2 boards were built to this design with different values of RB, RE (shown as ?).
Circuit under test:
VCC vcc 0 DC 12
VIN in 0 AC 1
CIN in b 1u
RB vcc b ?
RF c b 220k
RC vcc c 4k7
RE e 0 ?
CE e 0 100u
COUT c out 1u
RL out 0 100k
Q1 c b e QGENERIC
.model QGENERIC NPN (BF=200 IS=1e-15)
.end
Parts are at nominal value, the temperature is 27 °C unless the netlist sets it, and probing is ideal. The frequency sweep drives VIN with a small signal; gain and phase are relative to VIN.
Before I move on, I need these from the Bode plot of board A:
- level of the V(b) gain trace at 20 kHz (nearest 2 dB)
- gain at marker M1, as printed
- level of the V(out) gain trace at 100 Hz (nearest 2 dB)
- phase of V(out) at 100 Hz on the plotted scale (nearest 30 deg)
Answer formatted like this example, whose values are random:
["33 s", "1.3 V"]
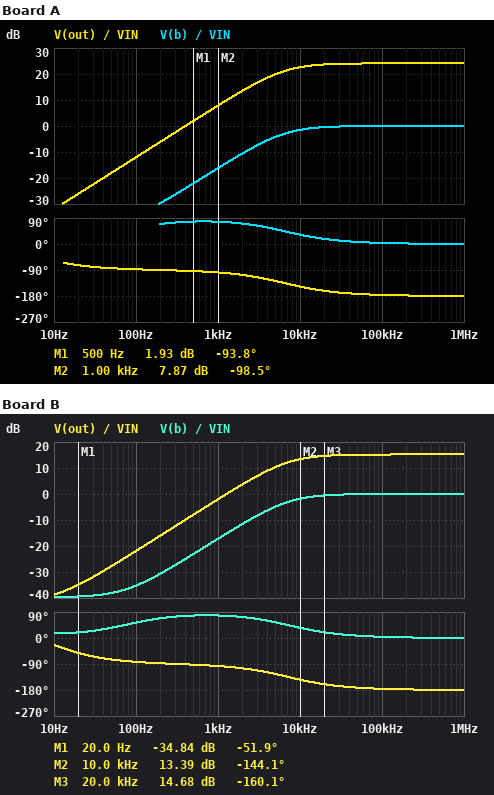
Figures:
["0 dB", "1.93 dB", "-12 dB", "-90 deg"]
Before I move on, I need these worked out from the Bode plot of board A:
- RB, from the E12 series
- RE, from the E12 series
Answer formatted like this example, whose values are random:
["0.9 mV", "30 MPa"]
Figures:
["120 kΩ", "1.2 kΩ"]
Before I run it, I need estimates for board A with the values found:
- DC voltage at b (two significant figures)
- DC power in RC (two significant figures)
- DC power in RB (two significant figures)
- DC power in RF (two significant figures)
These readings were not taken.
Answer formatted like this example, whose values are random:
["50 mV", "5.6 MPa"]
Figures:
["3.2 V", "19 mW", "640 µW", "1.9 µW"]
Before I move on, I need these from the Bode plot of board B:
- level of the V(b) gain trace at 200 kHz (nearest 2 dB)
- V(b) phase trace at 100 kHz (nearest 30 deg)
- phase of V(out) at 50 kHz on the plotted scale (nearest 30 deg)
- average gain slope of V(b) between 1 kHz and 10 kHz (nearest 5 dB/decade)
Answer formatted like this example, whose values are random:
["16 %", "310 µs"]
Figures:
["0 dB", "0 deg", "-180 deg", "15 dB/decade"]
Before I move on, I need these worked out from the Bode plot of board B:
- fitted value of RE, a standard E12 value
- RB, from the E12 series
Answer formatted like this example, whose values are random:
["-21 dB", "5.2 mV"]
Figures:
["1.2 kΩ", "47 kΩ"]
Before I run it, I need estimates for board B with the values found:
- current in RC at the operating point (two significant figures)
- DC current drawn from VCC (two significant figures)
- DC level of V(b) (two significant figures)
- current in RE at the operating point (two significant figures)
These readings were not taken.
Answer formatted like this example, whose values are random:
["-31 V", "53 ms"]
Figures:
["2.0 mA", "2.2 mA", "3.3 V", "2.2 mA"]
